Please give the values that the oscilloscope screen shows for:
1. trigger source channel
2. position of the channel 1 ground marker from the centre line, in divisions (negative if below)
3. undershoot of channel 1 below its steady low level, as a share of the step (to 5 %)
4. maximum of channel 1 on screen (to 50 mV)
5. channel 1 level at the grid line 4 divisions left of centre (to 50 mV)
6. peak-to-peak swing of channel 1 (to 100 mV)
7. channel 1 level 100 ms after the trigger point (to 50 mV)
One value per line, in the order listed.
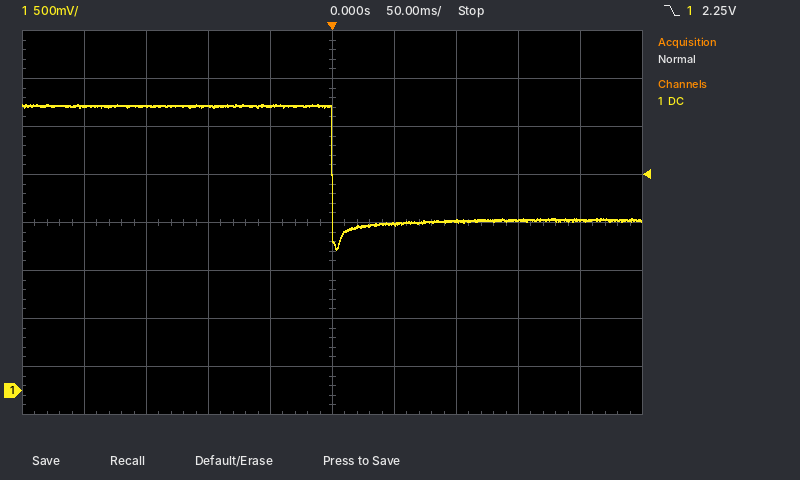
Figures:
channel 1
-3.5 div
25 %
3.00 V
2.95 V
1.50 V
1.75 V
